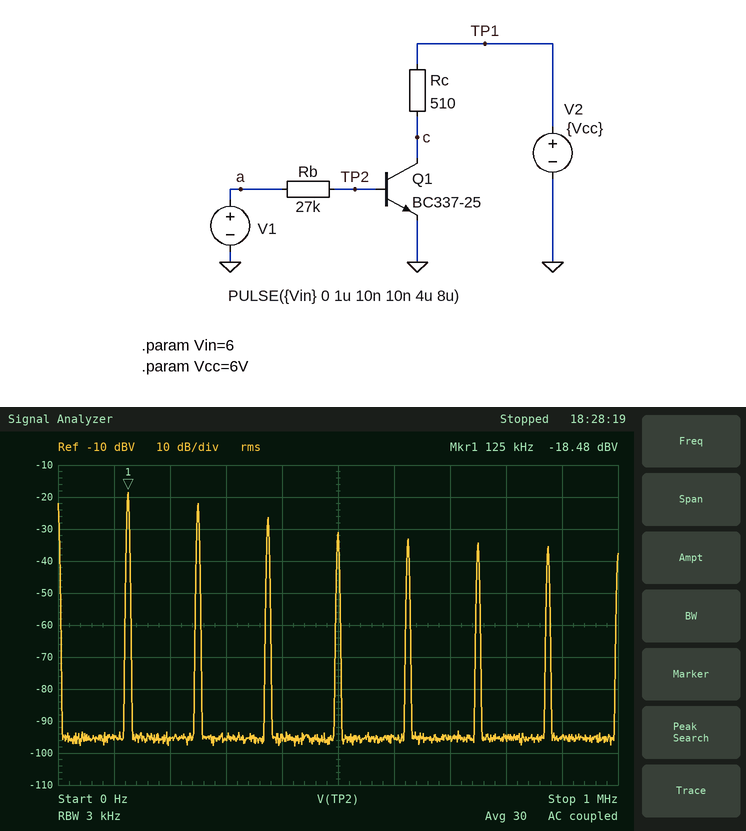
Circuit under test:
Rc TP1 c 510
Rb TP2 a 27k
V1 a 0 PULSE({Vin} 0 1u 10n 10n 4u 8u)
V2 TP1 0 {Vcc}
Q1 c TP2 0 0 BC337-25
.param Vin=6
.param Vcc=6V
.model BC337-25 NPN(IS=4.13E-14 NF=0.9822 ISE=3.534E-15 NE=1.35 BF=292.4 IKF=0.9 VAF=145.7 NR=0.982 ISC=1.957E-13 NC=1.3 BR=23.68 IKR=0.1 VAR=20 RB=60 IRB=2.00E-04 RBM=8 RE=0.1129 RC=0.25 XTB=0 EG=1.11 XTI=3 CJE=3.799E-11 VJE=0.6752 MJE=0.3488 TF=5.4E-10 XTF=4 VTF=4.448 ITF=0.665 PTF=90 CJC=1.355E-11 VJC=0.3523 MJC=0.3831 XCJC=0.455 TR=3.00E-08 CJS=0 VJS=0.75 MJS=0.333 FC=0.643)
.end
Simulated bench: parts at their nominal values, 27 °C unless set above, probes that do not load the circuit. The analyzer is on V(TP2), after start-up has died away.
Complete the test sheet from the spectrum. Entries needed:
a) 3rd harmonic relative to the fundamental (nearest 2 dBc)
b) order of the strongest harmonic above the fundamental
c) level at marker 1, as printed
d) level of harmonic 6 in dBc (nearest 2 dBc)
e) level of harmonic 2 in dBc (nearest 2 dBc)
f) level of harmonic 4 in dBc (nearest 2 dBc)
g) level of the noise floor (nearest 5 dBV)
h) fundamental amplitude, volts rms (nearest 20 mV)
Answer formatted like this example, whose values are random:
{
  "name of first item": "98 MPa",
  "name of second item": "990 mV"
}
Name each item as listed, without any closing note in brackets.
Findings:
{
  "3rd harmonic relative to the fundamental": "-8 dBc",
  "order of the strongest harmonic above the fundamental": "2",
  "level at marker 1, as printed": "-18.48 dBV",
  "level of harmonic 6 in dBc": "-16 dBc",
  "level of harmonic 2 in dBc": "-4 dBc",
  "level of harmonic 4 in dBc": "-12 dBc",
  "level of the noise floor": "-95 dBV",
  "fundamental amplitude, volts rms": "120 mV"
}
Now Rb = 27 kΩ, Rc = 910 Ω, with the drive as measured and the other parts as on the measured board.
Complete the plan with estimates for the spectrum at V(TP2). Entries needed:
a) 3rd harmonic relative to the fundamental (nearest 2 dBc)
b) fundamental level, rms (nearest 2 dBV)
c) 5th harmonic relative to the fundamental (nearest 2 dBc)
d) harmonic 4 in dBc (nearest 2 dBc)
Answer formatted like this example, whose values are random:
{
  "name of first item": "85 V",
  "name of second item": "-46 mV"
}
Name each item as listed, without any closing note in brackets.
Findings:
{
  "3rd harmonic relative to the fundamental": "-6 dBc",
  "fundamental level, rms": "-22 dBV",
  "5th harmonic relative to the fundamental": "-12 dBc",
  "harmonic 4 in dBc": "-10 dBc"
}
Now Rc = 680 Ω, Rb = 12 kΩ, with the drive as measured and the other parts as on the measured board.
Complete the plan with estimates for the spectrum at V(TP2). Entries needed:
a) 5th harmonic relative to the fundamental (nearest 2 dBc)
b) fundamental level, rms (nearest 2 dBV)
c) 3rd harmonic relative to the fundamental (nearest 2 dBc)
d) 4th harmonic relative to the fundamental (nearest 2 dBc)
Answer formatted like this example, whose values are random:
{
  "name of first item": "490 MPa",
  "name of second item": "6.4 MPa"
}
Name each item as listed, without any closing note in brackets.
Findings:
{
  "5th harmonic relative to the fundamental": "-16 dBc",
  "fundamental level, rms": "-14 dBV",
  "3rd harmonic relative to the fundamental": "-10 dBc",
  "4th harmonic relative to the fundamental": "-18 dBc"
}
